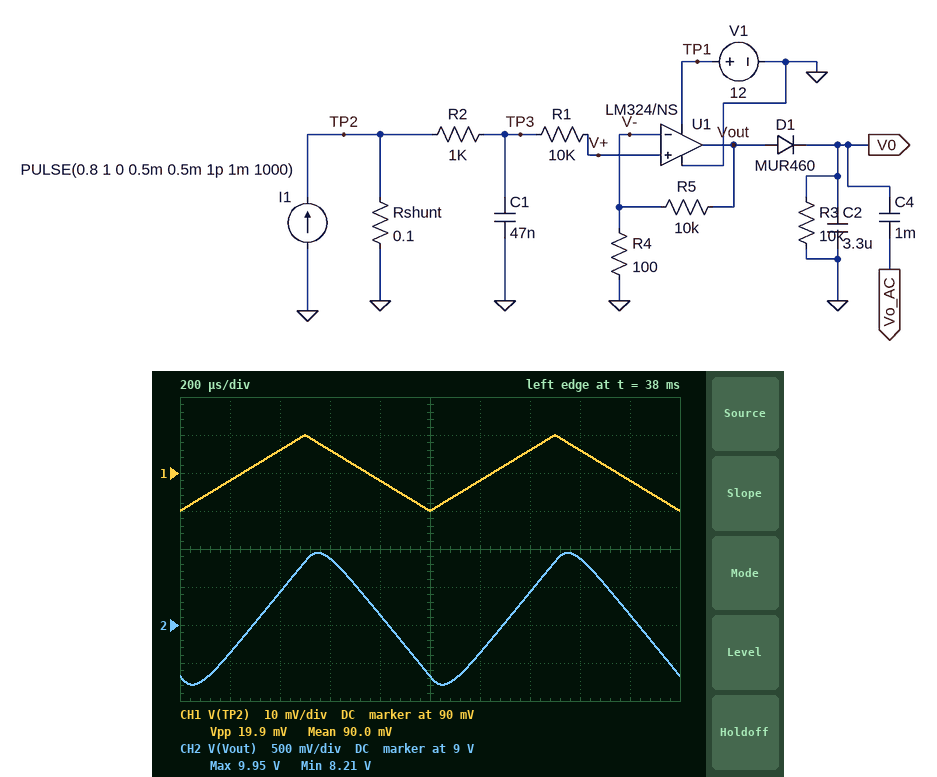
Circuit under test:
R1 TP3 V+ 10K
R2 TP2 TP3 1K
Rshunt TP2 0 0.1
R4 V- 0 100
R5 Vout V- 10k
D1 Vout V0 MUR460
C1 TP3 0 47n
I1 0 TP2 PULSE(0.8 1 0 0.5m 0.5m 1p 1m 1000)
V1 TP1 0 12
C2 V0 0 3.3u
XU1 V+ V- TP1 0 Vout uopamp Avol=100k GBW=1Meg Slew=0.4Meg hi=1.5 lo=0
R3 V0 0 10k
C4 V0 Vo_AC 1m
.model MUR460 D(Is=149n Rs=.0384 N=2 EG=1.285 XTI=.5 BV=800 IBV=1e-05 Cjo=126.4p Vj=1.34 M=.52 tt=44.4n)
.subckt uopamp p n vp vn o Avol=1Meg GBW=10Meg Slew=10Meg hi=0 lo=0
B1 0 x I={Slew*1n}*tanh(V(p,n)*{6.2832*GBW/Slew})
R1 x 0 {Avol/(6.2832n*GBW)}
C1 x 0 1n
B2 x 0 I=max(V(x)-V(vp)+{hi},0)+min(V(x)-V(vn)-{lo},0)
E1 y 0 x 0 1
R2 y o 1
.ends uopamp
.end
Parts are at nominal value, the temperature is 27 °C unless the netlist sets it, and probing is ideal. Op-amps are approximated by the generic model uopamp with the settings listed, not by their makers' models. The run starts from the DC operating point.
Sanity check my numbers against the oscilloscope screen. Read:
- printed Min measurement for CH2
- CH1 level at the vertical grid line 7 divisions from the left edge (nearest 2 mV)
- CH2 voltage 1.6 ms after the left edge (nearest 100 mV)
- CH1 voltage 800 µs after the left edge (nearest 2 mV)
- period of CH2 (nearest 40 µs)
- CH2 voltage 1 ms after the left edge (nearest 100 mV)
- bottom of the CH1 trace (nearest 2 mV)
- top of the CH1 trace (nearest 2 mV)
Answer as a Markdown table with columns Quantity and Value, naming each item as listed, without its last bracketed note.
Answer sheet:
| Quantity | Value |
|---|---|
| printed Min measurement for CH2 | 8.21 V |
| CH1 level at the vertical grid line 7 divisions from the left edge | 96 mV |
| CH2 voltage 1.6 ms after the left edge | 9.9 V |
| CH1 voltage 800 µs after the left edge | 88 mV |
| period of CH2 | 1.00 ms |
| CH2 voltage 1 ms after the left edge | 8.3 V |
| bottom of the CH1 trace | 80 mV |
| top of the CH1 trace | 100 mV |
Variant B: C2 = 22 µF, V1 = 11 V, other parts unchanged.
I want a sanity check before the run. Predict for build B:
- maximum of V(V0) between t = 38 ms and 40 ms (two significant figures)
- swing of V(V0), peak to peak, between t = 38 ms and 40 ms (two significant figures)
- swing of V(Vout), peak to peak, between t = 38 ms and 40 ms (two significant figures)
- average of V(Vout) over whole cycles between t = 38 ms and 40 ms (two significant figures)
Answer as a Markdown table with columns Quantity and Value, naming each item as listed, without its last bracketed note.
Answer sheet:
| Quantity | Value |
|---|---|
| maximum of V(V0) between t = 38 ms and 40 ms | 9.0 V |
| swing of V(V0), peak to peak, between t = 38 ms and 40 ms | 27 mV |
| swing of V(Vout), peak to peak, between t = 38 ms and 40 ms | 1.3 V |
| average of V(Vout) over whole cycles between t = 38 ms and 40 ms | 9.0 V |
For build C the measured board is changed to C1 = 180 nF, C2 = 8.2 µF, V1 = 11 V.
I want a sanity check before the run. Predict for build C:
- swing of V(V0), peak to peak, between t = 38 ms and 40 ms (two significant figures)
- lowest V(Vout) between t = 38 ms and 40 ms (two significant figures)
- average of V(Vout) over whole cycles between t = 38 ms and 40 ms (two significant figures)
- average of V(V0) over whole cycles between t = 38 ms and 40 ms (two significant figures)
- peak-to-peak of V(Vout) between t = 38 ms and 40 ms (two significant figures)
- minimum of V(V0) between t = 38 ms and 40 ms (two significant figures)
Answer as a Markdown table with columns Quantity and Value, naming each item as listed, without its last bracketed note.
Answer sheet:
| Quantity | Value |
|---|---|
| swing of V(V0), peak to peak, between t = 38 ms and 40 ms | 75 mV |
| lowest V(Vout) between t = 38 ms and 40 ms | 8.5 V |
| average of V(Vout) over whole cycles between t = 38 ms and 40 ms | 9.1 V |
| average of V(V0) over whole cycles between t = 38 ms and 40 ms | 9.0 V |
| peak-to-peak of V(Vout) between t = 38 ms and 40 ms | 960 mV |
| minimum of V(V0) between t = 38 ms and 40 ms | 8.9 V |
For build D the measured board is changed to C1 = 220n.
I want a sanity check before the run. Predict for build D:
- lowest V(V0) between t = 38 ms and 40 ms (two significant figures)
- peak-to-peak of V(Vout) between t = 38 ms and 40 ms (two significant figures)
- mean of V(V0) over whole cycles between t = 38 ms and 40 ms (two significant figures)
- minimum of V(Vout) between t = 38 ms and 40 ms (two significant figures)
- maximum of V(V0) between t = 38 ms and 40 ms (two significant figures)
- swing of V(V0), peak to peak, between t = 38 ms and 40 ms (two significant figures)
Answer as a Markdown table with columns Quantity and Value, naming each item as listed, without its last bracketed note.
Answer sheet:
| Quantity | Value |
|---|---|
| lowest V(V0) between t = 38 ms and 40 ms | 8.9 V |
| peak-to-peak of V(Vout) between t = 38 ms and 40 ms | 960 mV |
| mean of V(V0) over whole cycles between t = 38 ms and 40 ms | 9.0 V |
| minimum of V(Vout) between t = 38 ms and 40 ms | 8.6 V |
| maximum of V(V0) between t = 38 ms and 40 ms | 9.1 V |
| swing of V(V0), peak to peak, between t = 38 ms and 40 ms | 200 mV |
